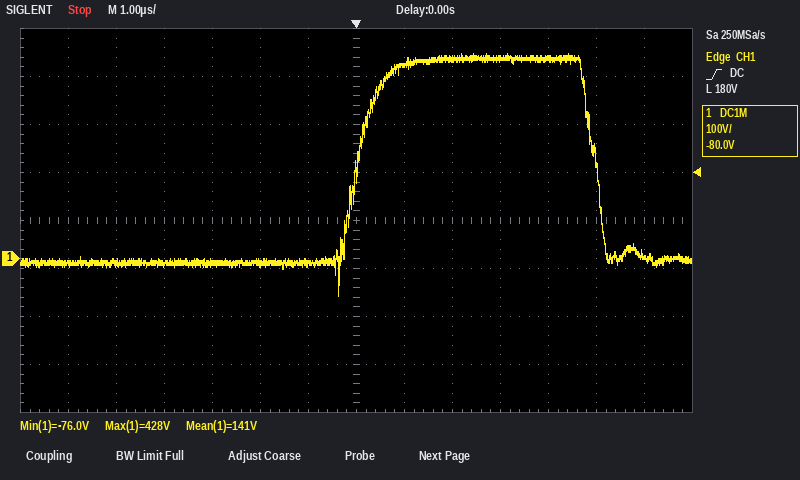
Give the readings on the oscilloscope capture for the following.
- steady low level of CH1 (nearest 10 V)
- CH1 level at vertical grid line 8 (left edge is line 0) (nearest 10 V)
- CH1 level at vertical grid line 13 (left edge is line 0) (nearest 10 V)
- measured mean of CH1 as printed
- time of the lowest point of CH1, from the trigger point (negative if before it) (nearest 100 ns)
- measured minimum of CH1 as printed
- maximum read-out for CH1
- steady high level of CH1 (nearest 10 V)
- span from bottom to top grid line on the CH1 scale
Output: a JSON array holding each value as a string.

["-10 V", "400 V", "10 V", "141 V", "-400 ns", "-76.0 V", "428 V", "420 V", "800 V"]
